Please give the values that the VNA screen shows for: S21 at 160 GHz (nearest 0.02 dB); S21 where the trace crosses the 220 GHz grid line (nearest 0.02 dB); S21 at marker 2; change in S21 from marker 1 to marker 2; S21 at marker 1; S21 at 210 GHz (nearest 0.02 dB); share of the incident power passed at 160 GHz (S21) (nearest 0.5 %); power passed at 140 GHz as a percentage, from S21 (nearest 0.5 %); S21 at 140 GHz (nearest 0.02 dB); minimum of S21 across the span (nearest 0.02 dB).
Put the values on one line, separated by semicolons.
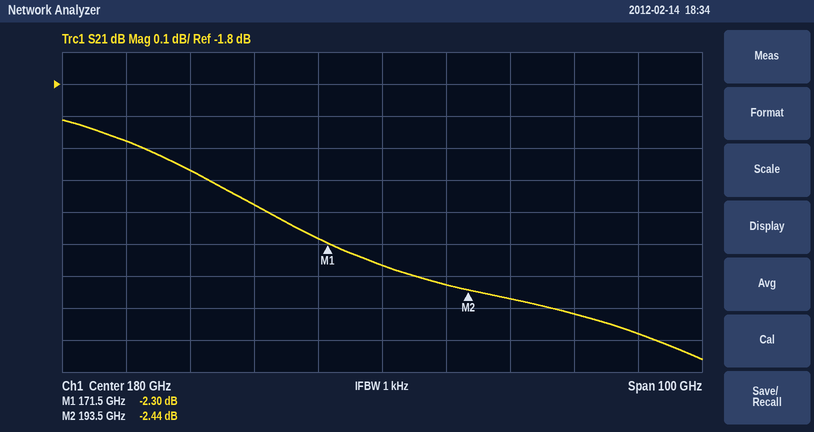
-2.18 dB; -2.58 dB; -2.44 dB; -0.14 dB; -2.30 dB; -2.52 dB; 60.5 %; 63.5 %; -1.98 dB; -2.66 dB
